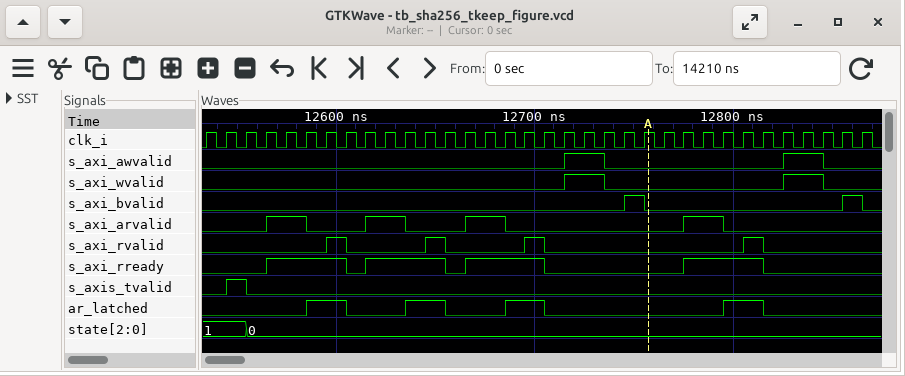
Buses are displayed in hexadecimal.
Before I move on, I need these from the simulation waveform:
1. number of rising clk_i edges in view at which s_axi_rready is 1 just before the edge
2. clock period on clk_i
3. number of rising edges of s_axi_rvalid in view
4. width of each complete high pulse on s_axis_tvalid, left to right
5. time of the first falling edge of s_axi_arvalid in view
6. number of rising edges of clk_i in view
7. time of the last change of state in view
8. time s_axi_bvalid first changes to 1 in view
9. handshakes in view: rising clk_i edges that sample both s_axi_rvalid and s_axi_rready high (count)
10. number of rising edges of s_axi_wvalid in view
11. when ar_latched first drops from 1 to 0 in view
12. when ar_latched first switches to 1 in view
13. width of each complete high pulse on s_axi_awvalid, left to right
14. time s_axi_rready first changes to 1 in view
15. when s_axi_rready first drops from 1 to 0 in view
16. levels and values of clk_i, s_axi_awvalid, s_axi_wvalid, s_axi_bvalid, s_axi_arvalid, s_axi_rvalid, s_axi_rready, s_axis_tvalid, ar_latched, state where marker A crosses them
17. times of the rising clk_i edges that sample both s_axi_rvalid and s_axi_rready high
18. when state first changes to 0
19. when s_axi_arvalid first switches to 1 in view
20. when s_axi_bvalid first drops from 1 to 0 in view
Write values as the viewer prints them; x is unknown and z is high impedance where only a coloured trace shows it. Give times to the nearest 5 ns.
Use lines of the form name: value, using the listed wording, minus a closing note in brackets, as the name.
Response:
number of rising clk_i edges in view at which s_axi_rready is 1 just before the edge: 16
clock period on clk_i: 10 ns
number of rising edges of s_axi_rvalid in view: 4
width of each complete high pulse on s_axis_tvalid, left to right: 10 ns
time of the first falling edge of s_axi_arvalid in view: 12585 ns
number of rising edges of clk_i in view: 34
time of the last change of state in view: 12555 ns
time s_axi_bvalid first changes to 1 in view: 12745 ns
handshakes in view: rising clk_i edges that sample both s_axi_rvalid and s_axi_rready high: 4
number of rising edges of s_axi_wvalid in view: 2
when ar_latched first drops from 1 to 0 in view: 12605 ns
when ar_latched first switches to 1 in view: 12585 ns
width of each complete high pulse on s_axi_awvalid, left to right: 20 ns, 20 ns
time s_axi_rready first changes to 1 in view: 12565 ns
when s_axi_rready first drops from 1 to 0 in view: 12605 ns
levels and values of clk_i, s_axi_awvalid, s_axi_wvalid, s_axi_bvalid, s_axi_arvalid, s_axi_rvalid, s_axi_rready, s_axis_tvalid, ar_latched, state where marker A crosses them: clk_i=1, s_axi_awvalid=0, s_axi_wvalid=0, s_axi_bvalid=0, s_axi_arvalid=0, s_axi_rvalid=0, s_axi_rready=0, s_axis_tvalid=0, ar_latched=0, state=0
times of the rising clk_i edges that sample both s_axi_rvalid and s_axi_rready high: 12605 ns, 12655 ns, 12705 ns, 12815 ns
when state first changes to 0: 12555 ns
when s_axi_arvalid first switches to 1 in view: 12565 ns
when s_axi_bvalid first drops from 1 to 0 in view: 12755 ns
